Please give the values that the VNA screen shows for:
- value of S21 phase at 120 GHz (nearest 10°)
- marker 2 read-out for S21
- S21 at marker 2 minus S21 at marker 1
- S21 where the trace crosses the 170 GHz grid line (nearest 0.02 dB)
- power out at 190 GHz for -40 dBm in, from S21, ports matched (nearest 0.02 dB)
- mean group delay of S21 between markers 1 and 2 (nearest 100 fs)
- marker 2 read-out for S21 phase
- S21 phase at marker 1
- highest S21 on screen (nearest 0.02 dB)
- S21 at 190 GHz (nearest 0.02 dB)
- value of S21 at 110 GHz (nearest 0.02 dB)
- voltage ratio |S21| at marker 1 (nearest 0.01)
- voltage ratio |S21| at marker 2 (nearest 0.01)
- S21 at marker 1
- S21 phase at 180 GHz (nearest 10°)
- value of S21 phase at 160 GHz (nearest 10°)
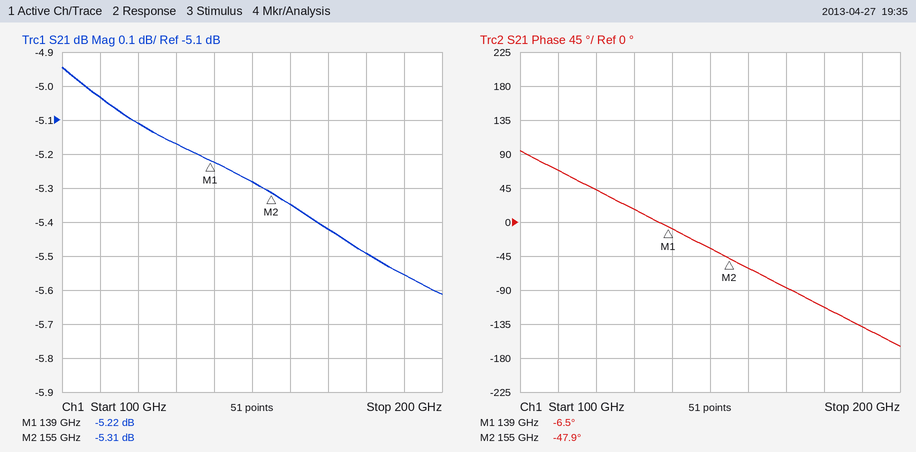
40°
-5.31 dB
-0.09 dB
-5.42 dB
-45.56 dBm
7.2 ps
-47.9°
-6.5°
-4.94 dB
-5.56 dB
-5.04 dB
0.55
0.54
-5.22 dB
-110°
-60°
